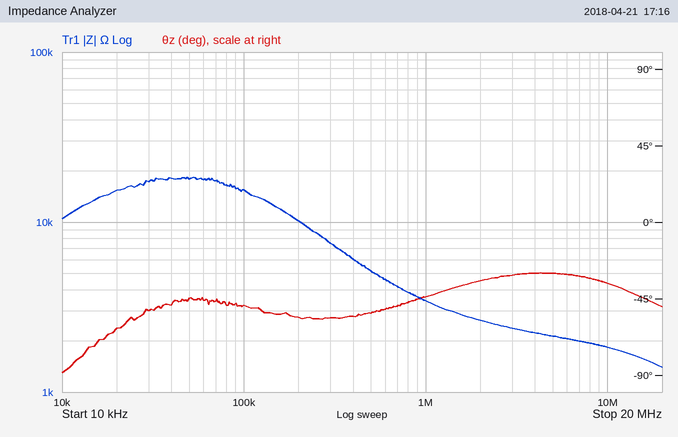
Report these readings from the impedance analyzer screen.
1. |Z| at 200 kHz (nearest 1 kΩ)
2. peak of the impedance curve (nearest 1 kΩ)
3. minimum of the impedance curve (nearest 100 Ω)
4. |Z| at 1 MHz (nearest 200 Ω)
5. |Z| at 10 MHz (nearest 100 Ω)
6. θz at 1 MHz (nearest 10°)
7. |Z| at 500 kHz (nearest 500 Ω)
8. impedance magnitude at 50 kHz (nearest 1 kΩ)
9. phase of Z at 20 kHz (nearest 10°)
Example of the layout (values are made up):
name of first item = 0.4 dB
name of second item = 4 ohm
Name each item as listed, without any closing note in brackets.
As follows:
|Z| at 200 kHz = 10 kΩ
peak of the impedance curve = 18 kΩ
minimum of the impedance curve = 1.4 kΩ
|Z| at 1 MHz = 3.4 kΩ
|Z| at 10 MHz = 1.8 kΩ
θz at 1 MHz = -40°
|Z| at 500 kHz = 5.0 kΩ
impedance magnitude at 50 kHz = 18 kΩ
phase of Z at 20 kHz = -60°
